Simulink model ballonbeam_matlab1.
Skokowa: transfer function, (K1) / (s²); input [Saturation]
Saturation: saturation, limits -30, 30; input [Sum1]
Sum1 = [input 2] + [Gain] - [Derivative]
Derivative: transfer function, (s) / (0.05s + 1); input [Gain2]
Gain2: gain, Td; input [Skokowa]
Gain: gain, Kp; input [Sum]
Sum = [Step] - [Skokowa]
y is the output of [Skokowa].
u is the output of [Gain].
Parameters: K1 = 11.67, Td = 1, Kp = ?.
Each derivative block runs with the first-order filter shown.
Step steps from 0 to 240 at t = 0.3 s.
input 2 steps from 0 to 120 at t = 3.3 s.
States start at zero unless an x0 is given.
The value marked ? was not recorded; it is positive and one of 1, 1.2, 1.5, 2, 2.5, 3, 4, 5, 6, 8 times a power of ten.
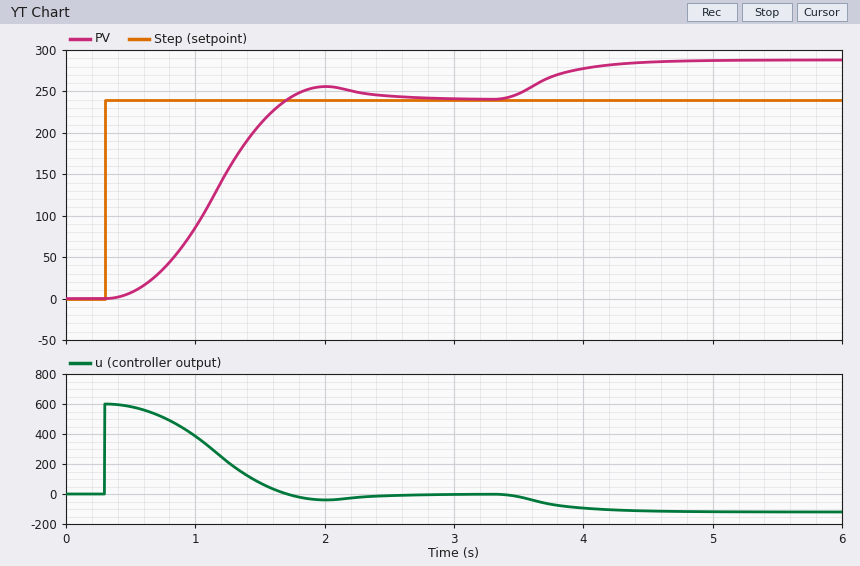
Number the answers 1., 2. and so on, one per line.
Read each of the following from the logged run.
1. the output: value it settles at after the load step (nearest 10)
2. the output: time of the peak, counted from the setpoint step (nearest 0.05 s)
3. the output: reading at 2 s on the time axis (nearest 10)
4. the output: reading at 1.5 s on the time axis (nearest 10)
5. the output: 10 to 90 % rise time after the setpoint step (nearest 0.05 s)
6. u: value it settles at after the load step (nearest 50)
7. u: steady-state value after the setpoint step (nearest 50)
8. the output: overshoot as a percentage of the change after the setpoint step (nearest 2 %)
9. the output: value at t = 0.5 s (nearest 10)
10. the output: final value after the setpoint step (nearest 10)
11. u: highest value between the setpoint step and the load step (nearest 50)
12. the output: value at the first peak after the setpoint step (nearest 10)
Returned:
1. 290
2. 1.70 s
3. 260
4. 210
5. 0.85 s
6. -100
7. 0
8. 6 %
9. 10
10. 240
11. 600
12. 260
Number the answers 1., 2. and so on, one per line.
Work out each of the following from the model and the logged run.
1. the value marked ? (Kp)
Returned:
1. 2.5
